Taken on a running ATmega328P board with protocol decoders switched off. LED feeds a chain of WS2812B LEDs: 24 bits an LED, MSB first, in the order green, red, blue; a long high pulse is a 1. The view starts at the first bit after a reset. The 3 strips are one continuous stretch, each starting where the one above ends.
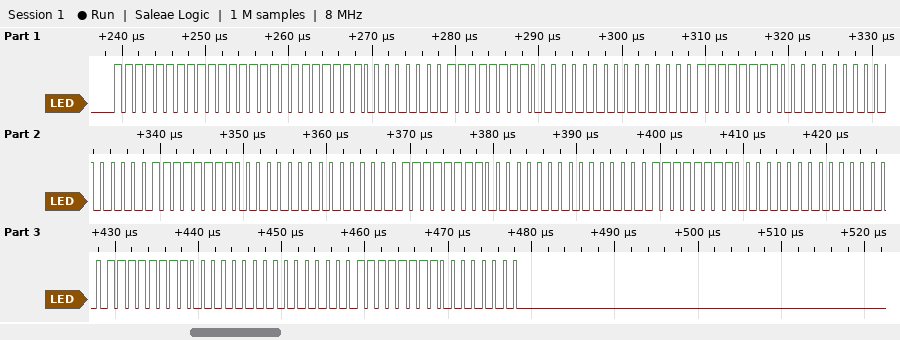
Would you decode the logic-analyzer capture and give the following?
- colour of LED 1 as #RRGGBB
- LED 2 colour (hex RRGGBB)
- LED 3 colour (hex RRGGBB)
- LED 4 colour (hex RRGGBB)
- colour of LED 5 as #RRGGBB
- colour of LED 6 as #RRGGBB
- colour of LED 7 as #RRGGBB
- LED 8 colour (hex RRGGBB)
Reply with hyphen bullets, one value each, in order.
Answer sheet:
- #FFFFFF
- #FF0000
- #FF0000
- #FF0000
- #FF0000
- #FF0000
- #FF0000
- #FF0000
